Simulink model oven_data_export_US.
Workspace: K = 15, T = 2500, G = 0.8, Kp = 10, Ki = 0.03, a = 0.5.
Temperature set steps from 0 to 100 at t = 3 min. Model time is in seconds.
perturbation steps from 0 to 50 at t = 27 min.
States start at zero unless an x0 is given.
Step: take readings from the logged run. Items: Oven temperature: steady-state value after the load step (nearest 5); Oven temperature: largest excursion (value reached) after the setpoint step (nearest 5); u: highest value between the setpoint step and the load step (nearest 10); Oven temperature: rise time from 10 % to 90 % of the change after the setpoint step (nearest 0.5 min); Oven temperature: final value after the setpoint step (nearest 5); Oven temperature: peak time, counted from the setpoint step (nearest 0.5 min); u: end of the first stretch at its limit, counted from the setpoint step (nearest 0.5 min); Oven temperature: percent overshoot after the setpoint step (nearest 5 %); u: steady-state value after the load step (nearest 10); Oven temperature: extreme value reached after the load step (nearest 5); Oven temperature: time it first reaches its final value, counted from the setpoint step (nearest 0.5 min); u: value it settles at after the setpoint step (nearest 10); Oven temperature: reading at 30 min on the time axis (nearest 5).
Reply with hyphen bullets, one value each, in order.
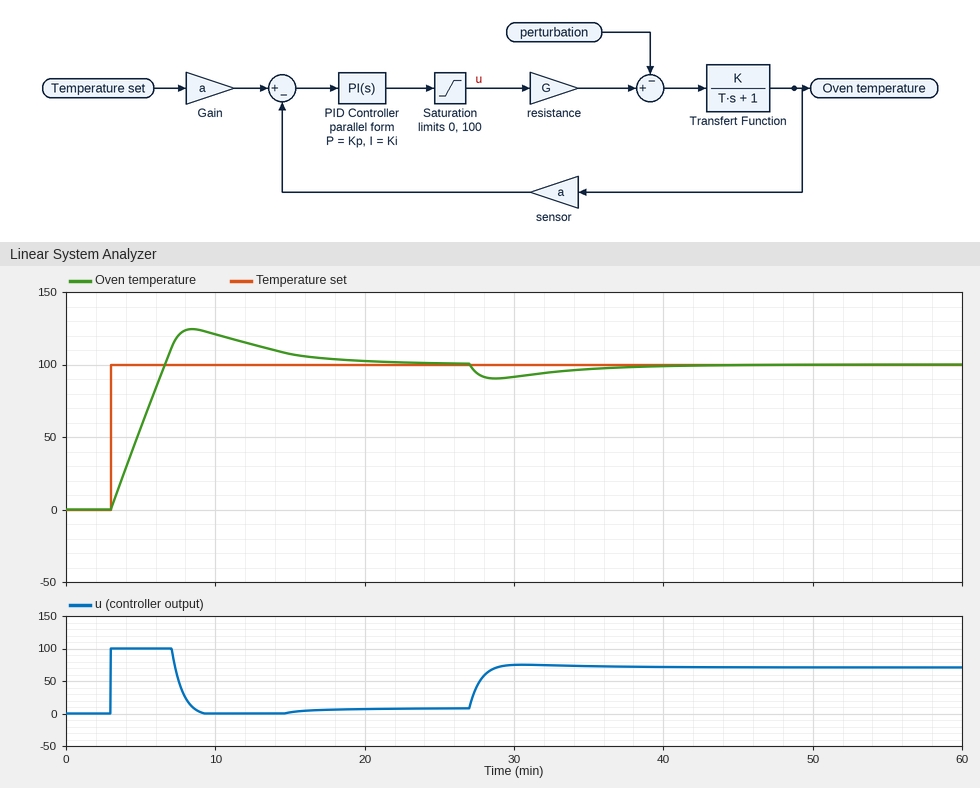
- 100
- 125
- 100
- 3.0 min
- 100
- 5.5 min
- 4.0 min
- 25 %
- 70
- 90
- 3.5 min
- 10
- 90
